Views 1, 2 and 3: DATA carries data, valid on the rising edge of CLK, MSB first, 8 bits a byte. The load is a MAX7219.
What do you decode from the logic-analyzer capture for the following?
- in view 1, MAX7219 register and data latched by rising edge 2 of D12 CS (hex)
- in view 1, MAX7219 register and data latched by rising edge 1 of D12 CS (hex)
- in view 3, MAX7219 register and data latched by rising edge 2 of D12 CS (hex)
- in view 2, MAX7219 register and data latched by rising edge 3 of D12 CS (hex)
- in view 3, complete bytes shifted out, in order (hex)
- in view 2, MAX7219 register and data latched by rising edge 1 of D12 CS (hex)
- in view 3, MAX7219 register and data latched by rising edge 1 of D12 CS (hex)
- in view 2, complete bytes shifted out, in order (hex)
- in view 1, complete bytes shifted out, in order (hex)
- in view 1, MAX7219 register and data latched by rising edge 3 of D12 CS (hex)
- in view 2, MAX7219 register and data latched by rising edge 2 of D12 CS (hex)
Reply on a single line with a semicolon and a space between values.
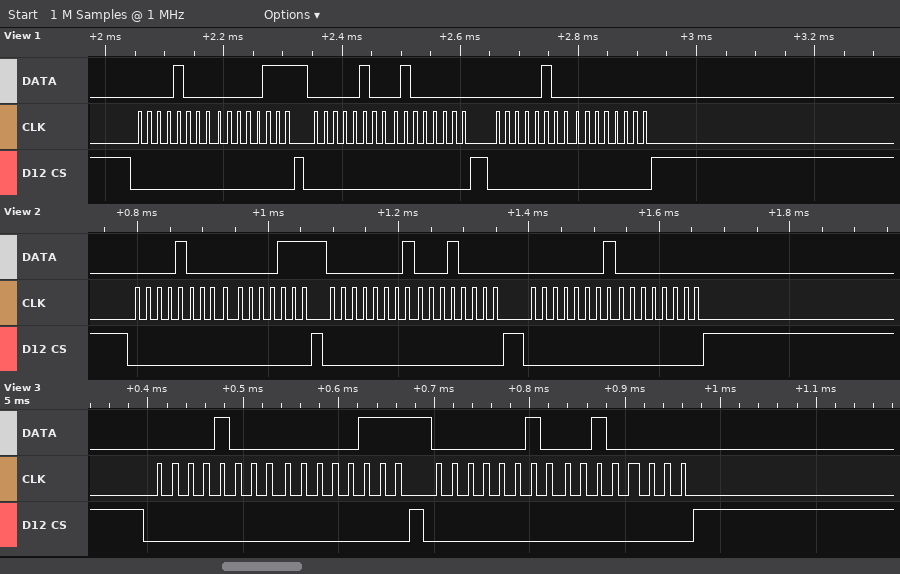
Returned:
register 0x4, data 0x40; register 0x8, data 0x07; register 0x2, data 0x20; register 0x1, data 0x00; 08 07 02 20; register 0x8, data 0x07; register 0x8, data 0x07; 0x08 0x07 0x01 0x10 0x01 0x00; 08 07 04 40 04 00; register 0x4, data 0x00; register 0x1, data 0x10
